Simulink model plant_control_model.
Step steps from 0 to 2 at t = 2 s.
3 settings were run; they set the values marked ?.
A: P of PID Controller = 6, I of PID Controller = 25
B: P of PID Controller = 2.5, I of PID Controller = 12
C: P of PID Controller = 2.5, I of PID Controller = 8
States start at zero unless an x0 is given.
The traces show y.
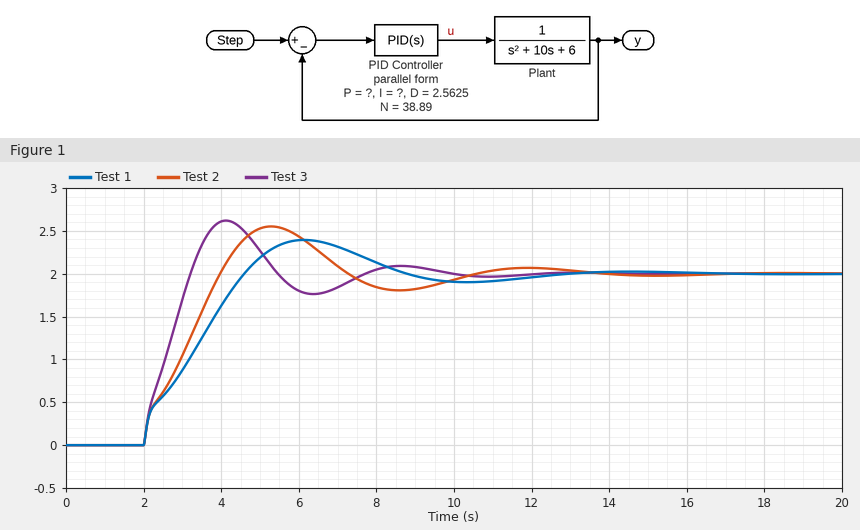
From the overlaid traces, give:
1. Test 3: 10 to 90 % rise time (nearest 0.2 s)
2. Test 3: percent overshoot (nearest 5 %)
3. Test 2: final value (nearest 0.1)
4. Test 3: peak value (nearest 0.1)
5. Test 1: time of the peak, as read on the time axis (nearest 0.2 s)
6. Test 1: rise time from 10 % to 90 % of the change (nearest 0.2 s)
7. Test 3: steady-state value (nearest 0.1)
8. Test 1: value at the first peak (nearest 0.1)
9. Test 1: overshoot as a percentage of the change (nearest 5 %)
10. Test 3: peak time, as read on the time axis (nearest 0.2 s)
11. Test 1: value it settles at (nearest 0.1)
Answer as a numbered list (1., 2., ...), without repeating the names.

1. 1.0 s
2. 30 %
3. 2.0
4. 2.6
5. 6.2 s
6. 2.2 s
7. 2.0
8. 2.4
9. 20 %
10. 4.2 s
11. 2.0
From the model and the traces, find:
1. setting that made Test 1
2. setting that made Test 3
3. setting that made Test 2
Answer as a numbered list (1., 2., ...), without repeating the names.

1. C
2. A
3. B
